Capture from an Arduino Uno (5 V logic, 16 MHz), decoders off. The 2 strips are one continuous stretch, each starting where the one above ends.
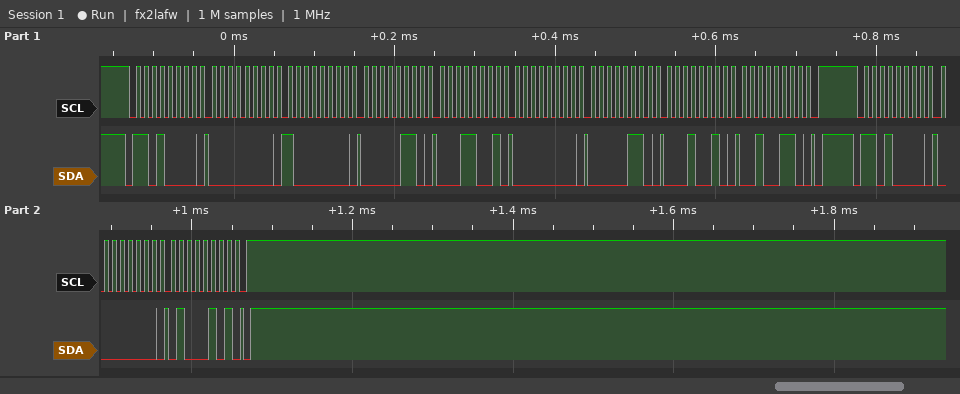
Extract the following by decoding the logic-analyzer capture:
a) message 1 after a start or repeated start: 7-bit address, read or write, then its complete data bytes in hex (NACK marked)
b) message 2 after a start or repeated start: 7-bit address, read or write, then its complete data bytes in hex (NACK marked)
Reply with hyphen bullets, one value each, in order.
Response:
- 0x68 write: 00 80 06 19 00 06 12 26
- 0x68 write: 00 45
